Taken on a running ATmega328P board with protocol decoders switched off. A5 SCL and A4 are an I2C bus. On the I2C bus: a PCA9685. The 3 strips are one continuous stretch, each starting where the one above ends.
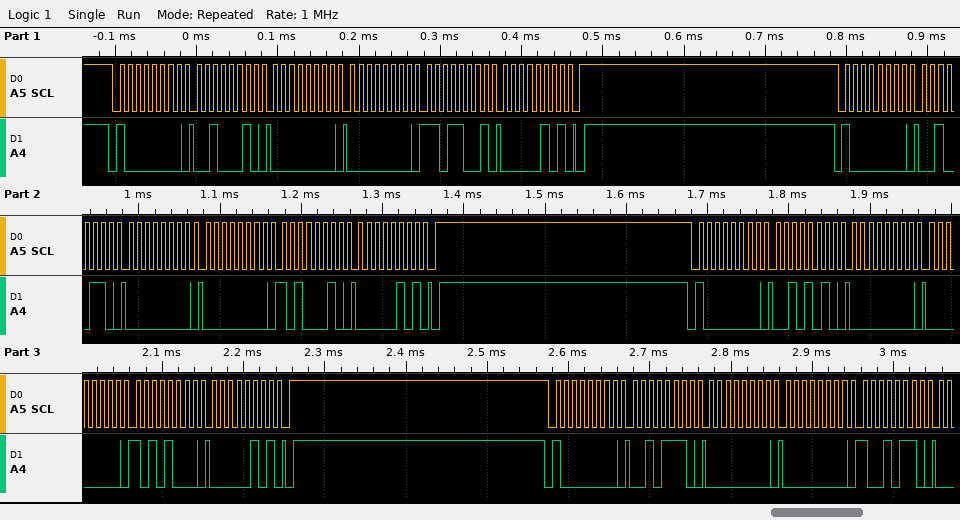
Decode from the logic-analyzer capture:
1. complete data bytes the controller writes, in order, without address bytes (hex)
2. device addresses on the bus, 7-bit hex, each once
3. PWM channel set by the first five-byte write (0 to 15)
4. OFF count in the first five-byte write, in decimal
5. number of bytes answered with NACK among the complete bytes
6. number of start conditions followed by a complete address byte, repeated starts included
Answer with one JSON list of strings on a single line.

["22 00 00 D9 05 26 00 00 A2 05 2A 00 00 A8 05 2E 00 00 96", "0x40", "7", "1497", "0", "4"]
